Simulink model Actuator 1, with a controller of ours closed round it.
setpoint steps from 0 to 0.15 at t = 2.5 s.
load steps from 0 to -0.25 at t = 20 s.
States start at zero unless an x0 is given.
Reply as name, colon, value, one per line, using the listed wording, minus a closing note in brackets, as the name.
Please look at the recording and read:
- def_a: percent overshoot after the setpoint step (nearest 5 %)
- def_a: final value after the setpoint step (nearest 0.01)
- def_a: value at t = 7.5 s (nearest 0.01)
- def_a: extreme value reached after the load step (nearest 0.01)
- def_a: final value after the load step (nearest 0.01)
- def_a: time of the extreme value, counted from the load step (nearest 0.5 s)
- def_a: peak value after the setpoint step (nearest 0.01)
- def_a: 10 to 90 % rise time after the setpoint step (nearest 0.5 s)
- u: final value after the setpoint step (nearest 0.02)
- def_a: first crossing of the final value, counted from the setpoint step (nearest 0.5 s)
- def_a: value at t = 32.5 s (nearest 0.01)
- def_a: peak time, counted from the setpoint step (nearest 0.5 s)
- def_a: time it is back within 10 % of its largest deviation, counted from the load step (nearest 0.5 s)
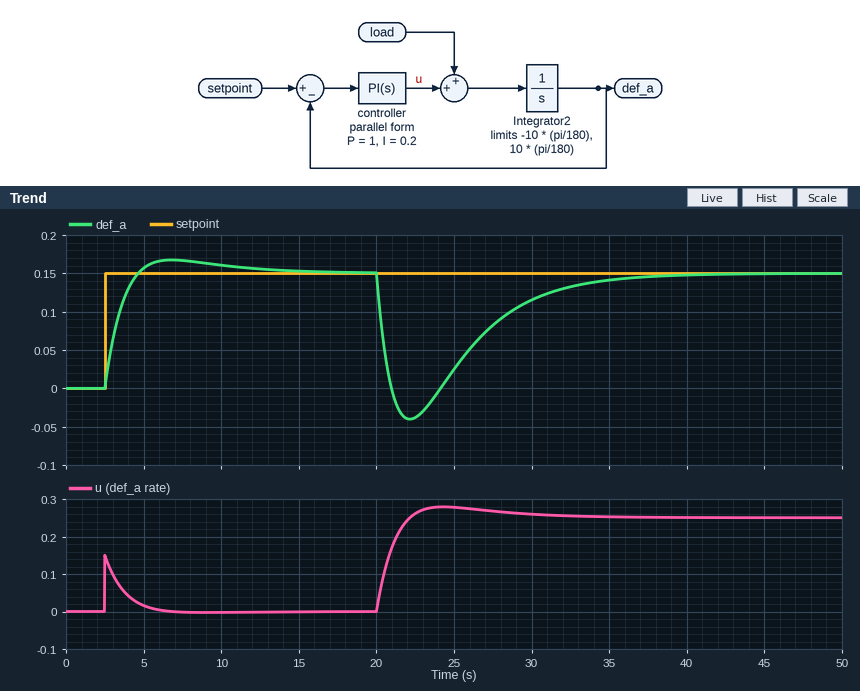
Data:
def_a: percent overshoot after the setpoint step: 10 %
def_a: final value after the setpoint step: 0.15
def_a: value at t = 7.5 s: 0.17
def_a: extreme value reached after the load step: -0.04
def_a: final value after the load step: 0.15
def_a: time of the extreme value, counted from the load step: 2.0 s
def_a: peak value after the setpoint step: 0.17
def_a: 10 to 90 % rise time after the setpoint step: 1.5 s
u: final value after the setpoint step: 0.00
def_a: first crossing of the final value, counted from the setpoint step: 2.0 s
def_a: value at t = 32.5 s: 0.13
def_a: peak time, counted from the setpoint step: 4.5 s
def_a: time it is back within 10 % of its largest deviation, counted from the load step: 12.0 s
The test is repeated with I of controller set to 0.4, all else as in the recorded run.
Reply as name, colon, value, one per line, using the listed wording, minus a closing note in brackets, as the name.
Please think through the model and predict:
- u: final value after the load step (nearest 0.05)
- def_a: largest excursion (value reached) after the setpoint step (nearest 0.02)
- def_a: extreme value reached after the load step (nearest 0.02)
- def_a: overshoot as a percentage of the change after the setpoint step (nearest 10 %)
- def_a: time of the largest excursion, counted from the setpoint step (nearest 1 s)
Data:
u: final value after the load step: 0.25
def_a: largest excursion (value reached) after the setpoint step: 0.18
def_a: extreme value reached after the load step: -0.02
def_a: overshoot as a percentage of the change after the setpoint step: 20 %
def_a: time of the largest excursion, counted from the setpoint step: 3 s
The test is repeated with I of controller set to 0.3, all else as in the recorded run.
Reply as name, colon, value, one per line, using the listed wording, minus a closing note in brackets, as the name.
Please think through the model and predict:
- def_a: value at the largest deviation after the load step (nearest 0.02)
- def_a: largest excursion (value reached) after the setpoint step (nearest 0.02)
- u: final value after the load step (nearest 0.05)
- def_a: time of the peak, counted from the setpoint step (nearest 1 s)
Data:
def_a: value at the largest deviation after the load step: -0.02
def_a: largest excursion (value reached) after the setpoint step: 0.18
u: final value after the load step: 0.25
def_a: time of the peak, counted from the setpoint step: 4 s
